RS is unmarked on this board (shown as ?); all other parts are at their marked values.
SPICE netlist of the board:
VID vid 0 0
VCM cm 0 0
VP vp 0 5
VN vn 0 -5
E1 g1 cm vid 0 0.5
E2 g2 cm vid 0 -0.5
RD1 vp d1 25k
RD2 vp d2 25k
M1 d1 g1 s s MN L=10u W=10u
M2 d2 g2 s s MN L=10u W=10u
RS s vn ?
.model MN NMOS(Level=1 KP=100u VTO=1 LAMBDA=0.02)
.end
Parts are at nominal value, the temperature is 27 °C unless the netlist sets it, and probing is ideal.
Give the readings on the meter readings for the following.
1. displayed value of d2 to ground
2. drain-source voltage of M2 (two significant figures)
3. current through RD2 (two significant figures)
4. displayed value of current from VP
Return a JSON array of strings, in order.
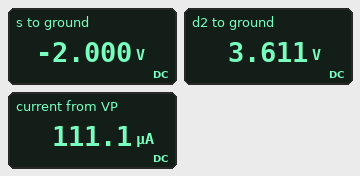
["3.611 V", "5.6 V", "56 µA", "111.1 µA"]
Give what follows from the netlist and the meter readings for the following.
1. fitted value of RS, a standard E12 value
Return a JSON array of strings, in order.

["27 kΩ"]
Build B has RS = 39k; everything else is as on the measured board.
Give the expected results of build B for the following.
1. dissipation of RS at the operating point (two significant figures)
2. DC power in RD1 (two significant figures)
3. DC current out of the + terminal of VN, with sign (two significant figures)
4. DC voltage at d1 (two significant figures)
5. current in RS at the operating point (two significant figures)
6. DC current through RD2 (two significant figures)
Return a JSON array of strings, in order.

["250 µW", "41 µW", "-81 µA", "4.0 V", "81 µA", "40 µA"]
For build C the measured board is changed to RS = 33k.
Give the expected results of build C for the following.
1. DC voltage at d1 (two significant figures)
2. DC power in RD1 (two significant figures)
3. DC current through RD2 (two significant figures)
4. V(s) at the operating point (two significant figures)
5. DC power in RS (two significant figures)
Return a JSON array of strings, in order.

["3.8 V", "55 µW", "47 µA", "-1.9 V", "290 µW"]
